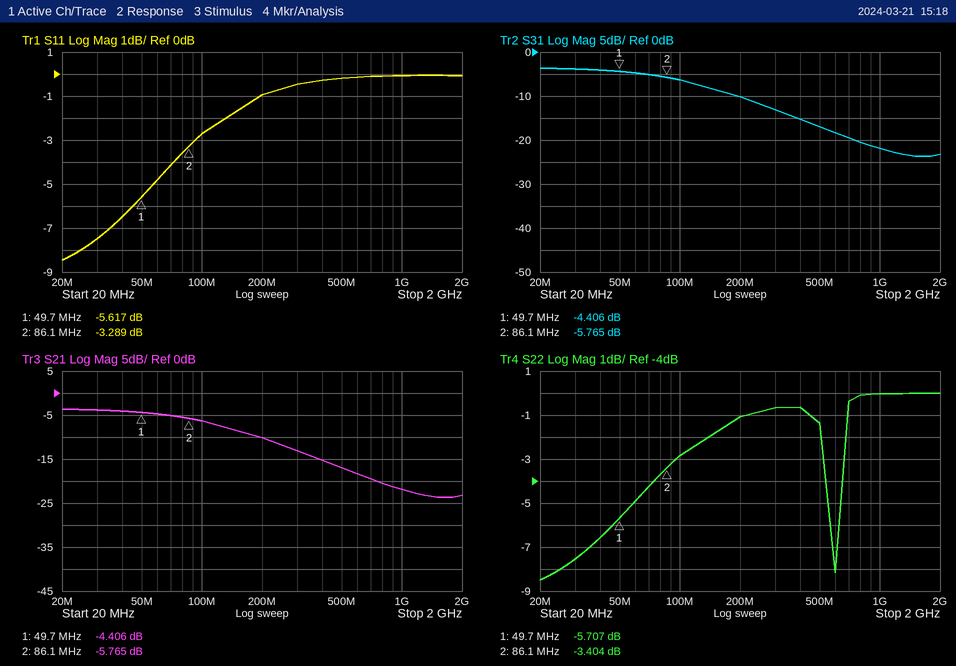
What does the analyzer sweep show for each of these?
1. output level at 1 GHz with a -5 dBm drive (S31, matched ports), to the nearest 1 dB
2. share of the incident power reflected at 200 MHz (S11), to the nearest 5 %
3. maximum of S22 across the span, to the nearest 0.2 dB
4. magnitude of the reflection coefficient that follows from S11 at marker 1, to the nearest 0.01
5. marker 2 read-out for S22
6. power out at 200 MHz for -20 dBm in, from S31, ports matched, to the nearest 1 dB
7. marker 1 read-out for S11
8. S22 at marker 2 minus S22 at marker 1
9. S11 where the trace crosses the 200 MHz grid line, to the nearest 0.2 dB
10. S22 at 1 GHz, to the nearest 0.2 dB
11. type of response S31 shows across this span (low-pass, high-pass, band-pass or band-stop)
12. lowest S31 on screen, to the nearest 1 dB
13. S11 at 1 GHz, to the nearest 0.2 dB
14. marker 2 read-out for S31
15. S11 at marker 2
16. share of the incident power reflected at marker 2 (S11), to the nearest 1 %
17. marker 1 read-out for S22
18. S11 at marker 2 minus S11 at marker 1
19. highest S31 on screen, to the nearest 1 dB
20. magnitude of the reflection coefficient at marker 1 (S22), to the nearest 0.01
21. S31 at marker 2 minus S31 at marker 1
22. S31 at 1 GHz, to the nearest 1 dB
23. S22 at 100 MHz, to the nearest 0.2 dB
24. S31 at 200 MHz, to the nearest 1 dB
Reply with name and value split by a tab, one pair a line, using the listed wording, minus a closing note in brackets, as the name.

output level at 1 GHz with a -5 dBm drive (S31, matched ports), to the nearest 1 dB	-27 dBm
share of the incident power reflected at 200 MHz (S11), to the nearest 5 %	80 %
maximum of S22 across the span, to the nearest 0.2 dB	0.0 dB
magnitude of the reflection coefficient that follows from S11 at marker 1, to the nearest 0.01	0.52
marker 2 read-out for S22	-3.404 dB
power out at 200 MHz for -20 dBm in, from S31, ports matched, to the nearest 1 dB	-30 dBm
marker 1 read-out for S11	-5.617 dB
S22 at marker 2 minus S22 at marker 1	2.303 dB
S11 where the trace crosses the 200 MHz grid line, to the nearest 0.2 dB	-1.0 dB
S22 at 1 GHz, to the nearest 0.2 dB	0.0 dB
type of response S31 shows across this span	low-pass
lowest S31 on screen, to the nearest 1 dB	-24 dB
S11 at 1 GHz, to the nearest 0.2 dB	0.0 dB
marker 2 read-out for S31	-5.765 dB
S11 at marker 2	-3.289 dB
share of the incident power reflected at marker 2 (S11), to the nearest 1 %	47 %
marker 1 read-out for S22	-5.707 dB
S11 at marker 2 minus S11 at marker 1	2.328 dB
highest S31 on screen, to the nearest 1 dB	-4 dB
magnitude of the reflection coefficient at marker 1 (S22), to the nearest 0.01	0.52
S31 at marker 2 minus S31 at marker 1	-1.359 dB
S31 at 1 GHz, to the nearest 1 dB	-22 dB
S22 at 100 MHz, to the nearest 0.2 dB	-2.8 dB
S31 at 200 MHz, to the nearest 1 dB	-10 dB
